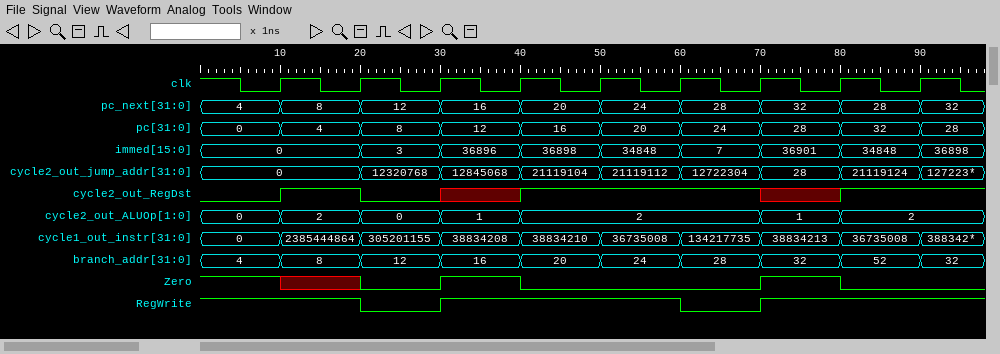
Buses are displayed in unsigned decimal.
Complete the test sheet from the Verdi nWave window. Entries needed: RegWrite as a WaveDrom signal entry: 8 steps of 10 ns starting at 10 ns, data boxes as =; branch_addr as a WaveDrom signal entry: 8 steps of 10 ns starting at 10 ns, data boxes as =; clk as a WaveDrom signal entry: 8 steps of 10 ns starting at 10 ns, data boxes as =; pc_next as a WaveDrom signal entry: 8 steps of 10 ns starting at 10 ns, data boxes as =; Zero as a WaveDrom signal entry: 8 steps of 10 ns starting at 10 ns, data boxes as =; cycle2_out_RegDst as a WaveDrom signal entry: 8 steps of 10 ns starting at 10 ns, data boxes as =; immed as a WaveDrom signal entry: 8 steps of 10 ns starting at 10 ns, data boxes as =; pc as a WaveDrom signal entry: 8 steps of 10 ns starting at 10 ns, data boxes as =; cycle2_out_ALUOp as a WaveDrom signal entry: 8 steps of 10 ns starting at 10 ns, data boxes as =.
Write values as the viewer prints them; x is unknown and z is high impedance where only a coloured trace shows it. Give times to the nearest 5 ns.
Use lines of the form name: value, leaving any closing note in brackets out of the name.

RegWrite as a WaveDrom signal entry: 8 steps of 10 ns starting at 10 ns, data boxes as =: {name: 'RegWrite', wave: '101..01.'}
branch_addr as a WaveDrom signal entry: 8 steps of 10 ns starting at 10 ns, data boxes as =: {name: 'branch_addr', wave: '========', data: '8 12 16 20 24 28 32 52'}
clk as a WaveDrom signal entry: 8 steps of 10 ns starting at 10 ns, data boxes as =: {name: 'clk', wave: 'p.......'}
pc_next as a WaveDrom signal entry: 8 steps of 10 ns starting at 10 ns, data boxes as =: {name: 'pc_next', wave: '========', data: '8 12 16 20 24 28 32 28'}
Zero as a WaveDrom signal entry: 8 steps of 10 ns starting at 10 ns, data boxes as =: {name: 'Zero', wave: 'x010..10'}
cycle2_out_RegDst as a WaveDrom signal entry: 8 steps of 10 ns starting at 10 ns, data boxes as =: {name: 'cycle2_out_RegDst', wave: '10x1..x1'}
immed as a WaveDrom signal entry: 8 steps of 10 ns starting at 10 ns, data boxes as =: {name: 'immed', wave: '========', data: '0 3 36896 36898 34848 7 36901 34848'}
pc as a WaveDrom signal entry: 8 steps of 10 ns starting at 10 ns, data boxes as =: {name: 'pc', wave: '========', data: '4 8 12 16 20 24 28 32'}
cycle2_out_ALUOp as a WaveDrom signal entry: 8 steps of 10 ns starting at 10 ns, data boxes as =: {name: 'cycle2_out_ALUOp', wave: '====..==', data: '2 0 1 2 1 2'}
